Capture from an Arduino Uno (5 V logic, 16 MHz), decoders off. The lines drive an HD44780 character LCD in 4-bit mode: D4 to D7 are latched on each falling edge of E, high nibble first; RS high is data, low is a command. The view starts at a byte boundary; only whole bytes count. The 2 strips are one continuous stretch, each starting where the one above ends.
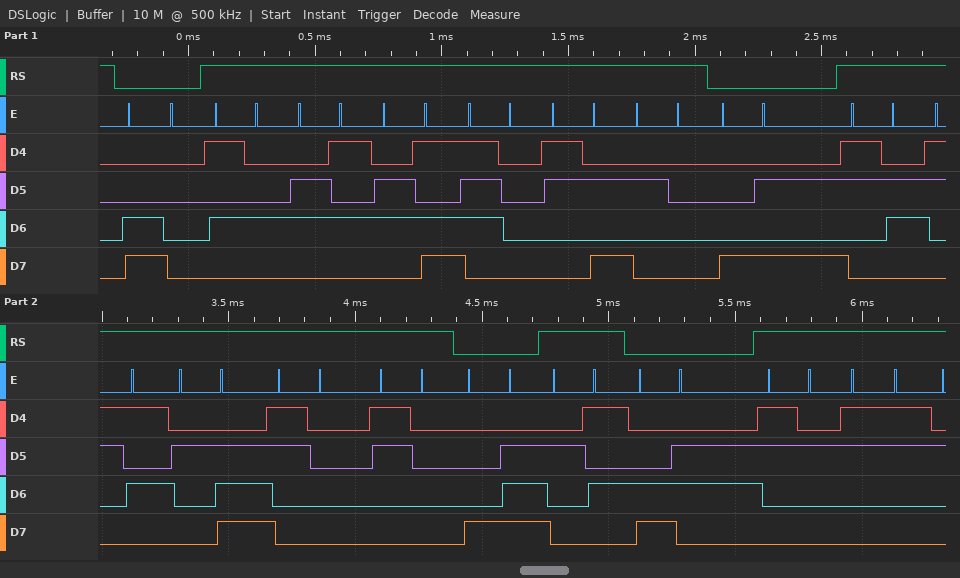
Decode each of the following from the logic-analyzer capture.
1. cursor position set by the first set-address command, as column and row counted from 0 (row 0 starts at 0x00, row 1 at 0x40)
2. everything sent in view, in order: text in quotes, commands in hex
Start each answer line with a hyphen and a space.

- column 0, row 1
- 0xC0 "Temp: " 0x8A "65.00" 0x8E "%" 0xC6 "23"
